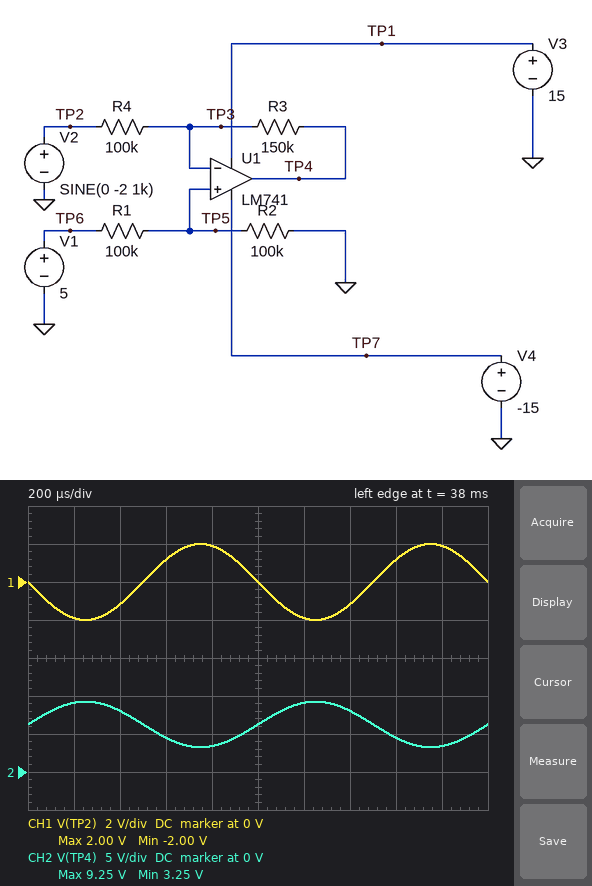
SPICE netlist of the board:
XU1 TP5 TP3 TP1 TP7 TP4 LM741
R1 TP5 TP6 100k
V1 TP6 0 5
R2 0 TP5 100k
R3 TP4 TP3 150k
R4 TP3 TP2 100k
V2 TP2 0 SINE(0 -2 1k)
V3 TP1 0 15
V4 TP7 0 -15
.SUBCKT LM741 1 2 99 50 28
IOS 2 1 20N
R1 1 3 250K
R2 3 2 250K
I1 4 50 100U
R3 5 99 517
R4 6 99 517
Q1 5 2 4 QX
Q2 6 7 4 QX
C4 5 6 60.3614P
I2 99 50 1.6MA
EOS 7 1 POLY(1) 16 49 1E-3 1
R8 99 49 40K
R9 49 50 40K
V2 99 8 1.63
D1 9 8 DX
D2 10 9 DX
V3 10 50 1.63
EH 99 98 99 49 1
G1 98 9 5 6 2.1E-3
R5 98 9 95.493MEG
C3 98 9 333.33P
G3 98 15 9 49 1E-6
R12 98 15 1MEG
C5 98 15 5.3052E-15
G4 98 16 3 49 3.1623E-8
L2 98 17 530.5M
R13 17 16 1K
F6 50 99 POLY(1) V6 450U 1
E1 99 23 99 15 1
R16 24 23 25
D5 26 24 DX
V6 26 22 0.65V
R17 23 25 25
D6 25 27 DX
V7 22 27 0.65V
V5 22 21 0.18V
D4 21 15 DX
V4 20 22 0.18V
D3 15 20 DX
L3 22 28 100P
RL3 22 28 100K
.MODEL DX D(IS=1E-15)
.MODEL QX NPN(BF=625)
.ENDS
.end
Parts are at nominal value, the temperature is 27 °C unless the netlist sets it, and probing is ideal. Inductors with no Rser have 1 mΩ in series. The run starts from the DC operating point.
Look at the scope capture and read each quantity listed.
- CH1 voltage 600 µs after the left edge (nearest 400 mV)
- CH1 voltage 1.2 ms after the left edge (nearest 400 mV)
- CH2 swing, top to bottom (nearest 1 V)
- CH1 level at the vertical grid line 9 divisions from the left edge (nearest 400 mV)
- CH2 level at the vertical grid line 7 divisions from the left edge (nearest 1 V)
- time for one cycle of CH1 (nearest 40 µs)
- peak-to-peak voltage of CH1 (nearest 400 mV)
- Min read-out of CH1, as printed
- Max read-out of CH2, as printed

1.2 V
-2.0 V
6 V
2.0 V
8 V
1.00 ms
4.0 V
-2.00 V
9.25 V
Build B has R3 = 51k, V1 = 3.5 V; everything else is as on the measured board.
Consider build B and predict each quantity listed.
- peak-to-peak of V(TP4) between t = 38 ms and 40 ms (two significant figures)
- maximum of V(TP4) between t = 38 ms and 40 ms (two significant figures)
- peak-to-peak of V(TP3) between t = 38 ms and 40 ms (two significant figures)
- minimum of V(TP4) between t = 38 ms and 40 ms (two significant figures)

2.0 V
3.7 V
2.4 mV
1.6 V
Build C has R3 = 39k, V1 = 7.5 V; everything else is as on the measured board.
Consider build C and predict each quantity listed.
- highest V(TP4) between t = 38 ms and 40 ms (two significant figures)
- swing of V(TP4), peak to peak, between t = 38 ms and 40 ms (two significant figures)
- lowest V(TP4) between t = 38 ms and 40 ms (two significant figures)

6.0 V
1.6 V
4.4 V
